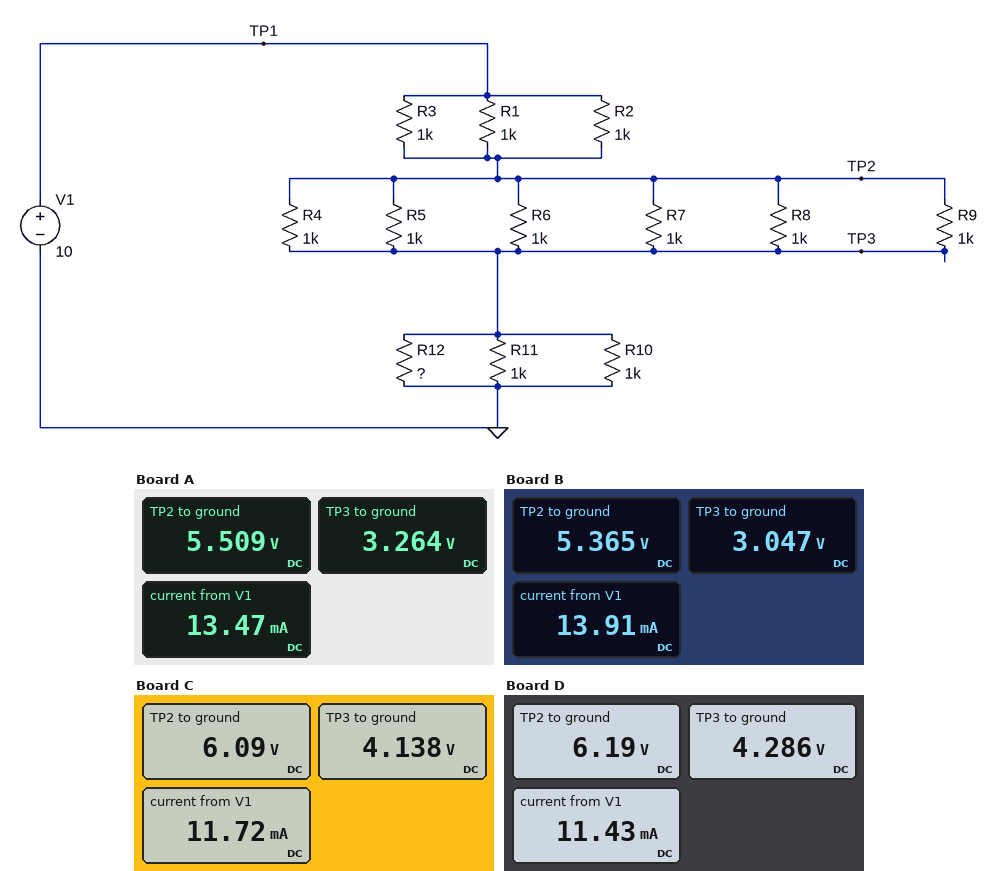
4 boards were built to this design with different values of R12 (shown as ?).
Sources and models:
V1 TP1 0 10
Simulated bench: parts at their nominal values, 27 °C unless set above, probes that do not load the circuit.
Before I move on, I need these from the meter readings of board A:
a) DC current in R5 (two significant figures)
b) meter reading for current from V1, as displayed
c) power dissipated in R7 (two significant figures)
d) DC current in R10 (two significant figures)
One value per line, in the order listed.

2.2 mA
13.47 mA
5.0 mW
3.3 mA
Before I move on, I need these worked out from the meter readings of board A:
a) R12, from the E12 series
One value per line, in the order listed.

470 Ω
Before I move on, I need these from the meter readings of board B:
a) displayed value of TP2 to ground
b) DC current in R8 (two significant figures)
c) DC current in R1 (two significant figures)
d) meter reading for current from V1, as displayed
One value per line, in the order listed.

5.365 V
2.3 mA
4.6 mA
13.91 mA
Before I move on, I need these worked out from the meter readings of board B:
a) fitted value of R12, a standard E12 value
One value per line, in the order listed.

390 Ω
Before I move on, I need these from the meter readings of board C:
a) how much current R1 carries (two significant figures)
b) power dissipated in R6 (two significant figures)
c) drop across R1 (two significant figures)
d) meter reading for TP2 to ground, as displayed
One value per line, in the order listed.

3.9 mA
3.8 mW
3.9 V
6.09 V
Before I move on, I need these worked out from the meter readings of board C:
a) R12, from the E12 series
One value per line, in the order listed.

1.2 kΩ
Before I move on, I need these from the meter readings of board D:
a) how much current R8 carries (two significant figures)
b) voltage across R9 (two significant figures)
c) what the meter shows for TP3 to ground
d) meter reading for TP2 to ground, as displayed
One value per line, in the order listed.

1.9 mA
1.9 V
4.286 V
6.19 V
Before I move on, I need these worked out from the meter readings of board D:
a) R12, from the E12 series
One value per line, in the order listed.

1.5 kΩ
